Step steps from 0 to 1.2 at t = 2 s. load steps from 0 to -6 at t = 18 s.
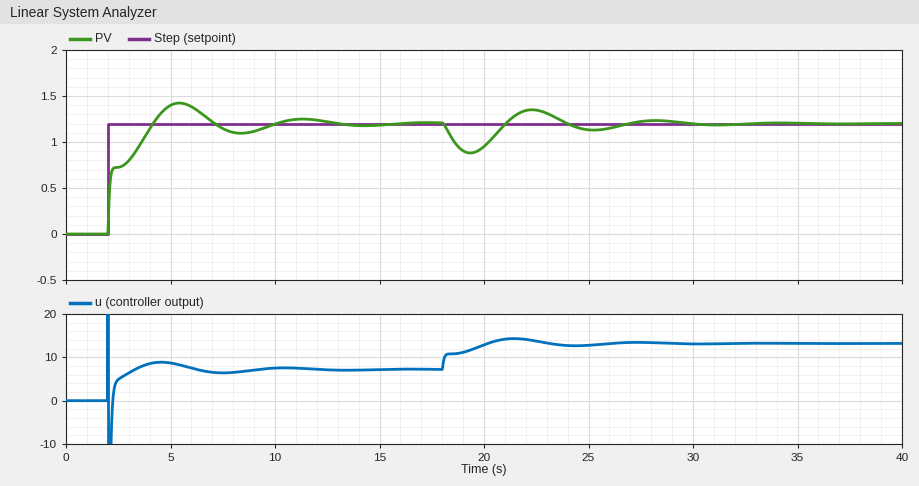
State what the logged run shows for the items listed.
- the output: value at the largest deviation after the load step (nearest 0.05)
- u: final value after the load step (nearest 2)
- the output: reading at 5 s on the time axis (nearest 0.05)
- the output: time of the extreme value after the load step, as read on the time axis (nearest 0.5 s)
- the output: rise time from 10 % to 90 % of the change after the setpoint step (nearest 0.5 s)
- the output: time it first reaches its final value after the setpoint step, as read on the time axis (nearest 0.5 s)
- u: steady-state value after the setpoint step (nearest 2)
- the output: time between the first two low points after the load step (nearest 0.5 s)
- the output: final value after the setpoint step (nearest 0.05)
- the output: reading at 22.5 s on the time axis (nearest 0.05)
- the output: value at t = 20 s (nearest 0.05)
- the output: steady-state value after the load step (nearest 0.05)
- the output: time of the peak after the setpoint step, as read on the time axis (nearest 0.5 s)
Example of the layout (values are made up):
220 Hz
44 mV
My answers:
0.90
14
1.40
19.5 s
2.0 s
4.0 s
8
6.0 s
1.20
1.35
0.95
1.20
5.5 s
